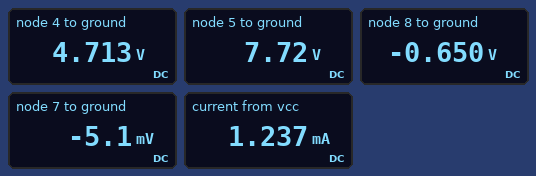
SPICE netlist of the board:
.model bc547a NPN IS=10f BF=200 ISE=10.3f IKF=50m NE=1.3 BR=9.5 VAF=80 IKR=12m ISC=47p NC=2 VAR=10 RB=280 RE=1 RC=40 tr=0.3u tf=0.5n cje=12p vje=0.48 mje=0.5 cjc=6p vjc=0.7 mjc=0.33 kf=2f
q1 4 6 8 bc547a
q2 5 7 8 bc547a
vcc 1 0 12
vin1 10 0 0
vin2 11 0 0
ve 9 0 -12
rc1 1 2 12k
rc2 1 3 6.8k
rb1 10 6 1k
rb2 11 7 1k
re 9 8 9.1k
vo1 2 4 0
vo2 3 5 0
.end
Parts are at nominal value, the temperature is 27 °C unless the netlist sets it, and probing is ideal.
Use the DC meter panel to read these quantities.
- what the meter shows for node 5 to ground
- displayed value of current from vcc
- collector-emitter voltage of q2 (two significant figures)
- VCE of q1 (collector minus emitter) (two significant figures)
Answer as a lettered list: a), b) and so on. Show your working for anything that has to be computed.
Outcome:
a) 7.72 V
b) 1.237 mA
c) 7.72 V - (-650 mV) = 8.4 V
d) 4.713 V - (-650 mV) = 5.4 V
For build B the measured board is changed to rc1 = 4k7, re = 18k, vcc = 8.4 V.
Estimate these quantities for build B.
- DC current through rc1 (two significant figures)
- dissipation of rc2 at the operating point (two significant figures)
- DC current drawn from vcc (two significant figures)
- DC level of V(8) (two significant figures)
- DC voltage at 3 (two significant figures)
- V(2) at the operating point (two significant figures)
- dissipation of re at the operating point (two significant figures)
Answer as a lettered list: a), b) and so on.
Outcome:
a) 310 µA
b) 660 µW
c) 630 µA
d) -630 mV
e) 6.3 V
f) 6.9 V
g) 7.2 mW
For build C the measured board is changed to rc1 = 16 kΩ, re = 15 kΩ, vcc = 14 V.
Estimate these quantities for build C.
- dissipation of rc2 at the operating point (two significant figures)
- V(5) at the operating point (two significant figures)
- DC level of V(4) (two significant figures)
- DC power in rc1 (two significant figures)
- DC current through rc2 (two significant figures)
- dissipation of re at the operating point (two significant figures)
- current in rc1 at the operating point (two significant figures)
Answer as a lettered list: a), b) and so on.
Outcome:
a) 1.0 mW
b) 11 V
c) 8.1 V
d) 2.2 mW
e) 380 µA
f) 8.6 mW
g) 370 µA
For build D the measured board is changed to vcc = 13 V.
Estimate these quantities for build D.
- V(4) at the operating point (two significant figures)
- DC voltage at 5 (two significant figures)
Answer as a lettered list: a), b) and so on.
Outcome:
a) 5.7 V
b) 8.7 V
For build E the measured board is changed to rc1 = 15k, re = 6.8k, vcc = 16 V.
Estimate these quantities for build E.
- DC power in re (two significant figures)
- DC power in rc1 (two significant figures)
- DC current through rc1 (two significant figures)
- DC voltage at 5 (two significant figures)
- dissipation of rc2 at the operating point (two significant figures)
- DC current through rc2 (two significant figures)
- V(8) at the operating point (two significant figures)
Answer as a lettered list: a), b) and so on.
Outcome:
a) 19 mW
b) 9.5 mW
c) 800 µA
d) 10 V
e) 5.0 mW
f) 860 µA
g) -660 mV
